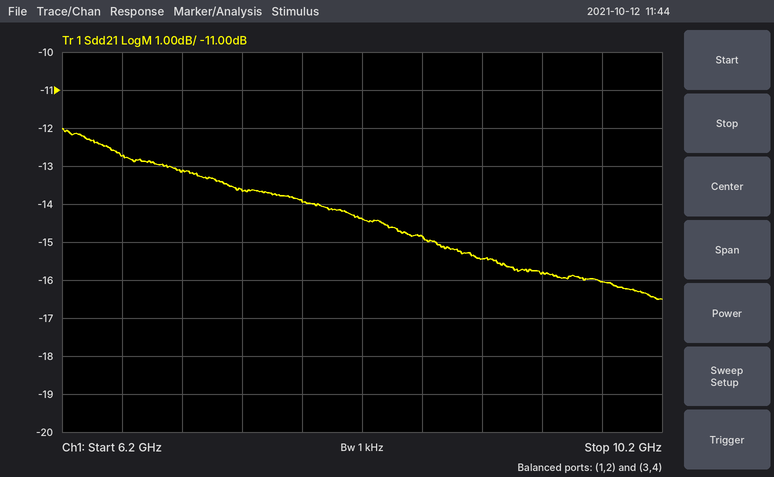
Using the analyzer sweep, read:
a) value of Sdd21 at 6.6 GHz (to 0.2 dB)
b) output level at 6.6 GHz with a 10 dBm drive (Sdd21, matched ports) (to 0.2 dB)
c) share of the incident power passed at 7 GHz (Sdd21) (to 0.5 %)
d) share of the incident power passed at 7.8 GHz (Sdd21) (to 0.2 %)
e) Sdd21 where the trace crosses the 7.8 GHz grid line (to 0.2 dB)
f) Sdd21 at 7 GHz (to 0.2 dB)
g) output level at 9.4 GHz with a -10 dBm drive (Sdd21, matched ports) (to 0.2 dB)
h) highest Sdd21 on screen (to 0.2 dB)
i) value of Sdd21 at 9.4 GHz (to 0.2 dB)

-12.8 dB
-2.8 dBm
5.0 %
4.0 %
-14.0 dB
-13.2 dB
-25.8 dBm
-12.0 dB
-15.8 dB
